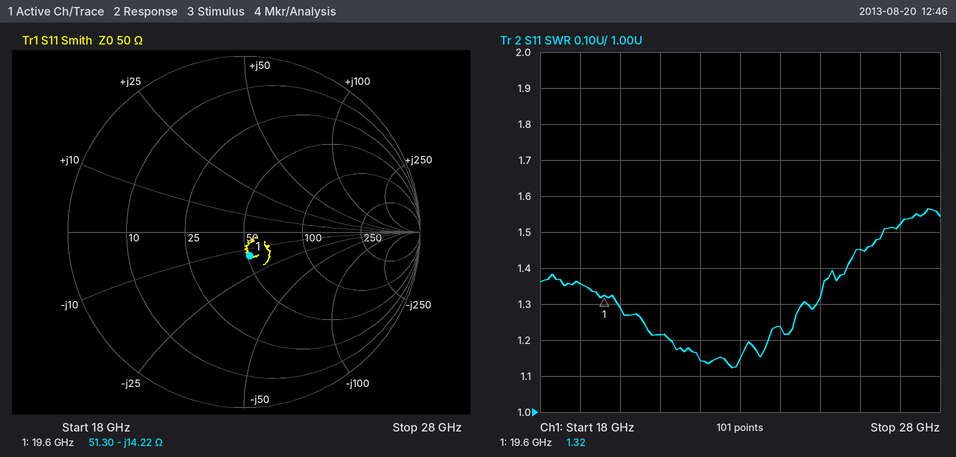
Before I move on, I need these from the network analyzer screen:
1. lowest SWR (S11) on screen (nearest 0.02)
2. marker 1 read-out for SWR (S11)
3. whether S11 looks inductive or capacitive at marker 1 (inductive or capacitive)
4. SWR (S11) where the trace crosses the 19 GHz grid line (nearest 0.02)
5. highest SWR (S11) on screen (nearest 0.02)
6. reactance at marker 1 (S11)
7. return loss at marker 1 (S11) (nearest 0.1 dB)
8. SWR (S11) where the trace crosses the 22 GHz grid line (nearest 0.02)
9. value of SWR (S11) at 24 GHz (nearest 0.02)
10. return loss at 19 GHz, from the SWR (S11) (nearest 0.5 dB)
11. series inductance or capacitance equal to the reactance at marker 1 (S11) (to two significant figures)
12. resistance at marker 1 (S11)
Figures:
1.12
1.32
capacitive
1.36
1.56
-14.22 Ω
17.1 dB
1.14
1.24
16.5 dB
570 fF
51.30 Ω
